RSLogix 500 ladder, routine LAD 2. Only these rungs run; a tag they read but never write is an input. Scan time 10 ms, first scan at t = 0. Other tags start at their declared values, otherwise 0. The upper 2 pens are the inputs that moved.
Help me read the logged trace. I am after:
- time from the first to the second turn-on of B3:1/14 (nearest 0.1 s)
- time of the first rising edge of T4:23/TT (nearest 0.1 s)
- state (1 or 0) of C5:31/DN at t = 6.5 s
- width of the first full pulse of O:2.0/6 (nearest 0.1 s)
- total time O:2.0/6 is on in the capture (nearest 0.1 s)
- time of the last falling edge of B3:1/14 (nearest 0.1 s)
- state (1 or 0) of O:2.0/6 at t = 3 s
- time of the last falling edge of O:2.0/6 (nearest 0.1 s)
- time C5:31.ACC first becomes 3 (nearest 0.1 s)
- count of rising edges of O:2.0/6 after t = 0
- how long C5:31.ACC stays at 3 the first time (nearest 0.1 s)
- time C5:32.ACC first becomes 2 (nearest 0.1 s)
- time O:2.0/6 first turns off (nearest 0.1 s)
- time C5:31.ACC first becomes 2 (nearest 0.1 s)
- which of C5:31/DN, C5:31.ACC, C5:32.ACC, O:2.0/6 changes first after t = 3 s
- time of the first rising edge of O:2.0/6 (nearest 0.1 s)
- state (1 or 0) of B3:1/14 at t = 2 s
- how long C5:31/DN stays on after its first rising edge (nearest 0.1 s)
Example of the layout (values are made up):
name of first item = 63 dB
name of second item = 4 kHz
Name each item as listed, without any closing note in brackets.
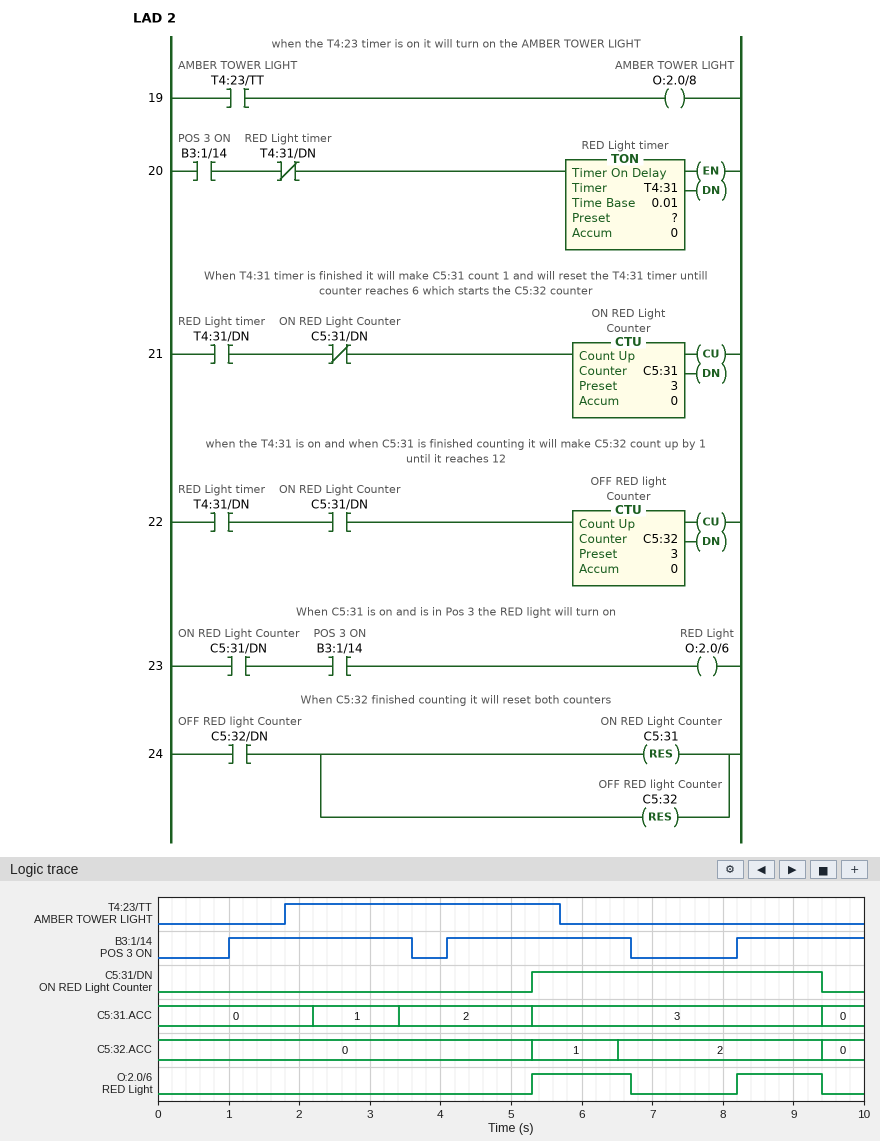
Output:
time from the first to the second turn-on of B3:1/14 = 3.1 s
time of the first rising edge of T4:23/TT = 1.8 s
state (1 or 0) of C5:31/DN at t = 6.5 s = 1
width of the first full pulse of O:2.0/6 = 1.4 s
total time O:2.0/6 is on in the capture = 2.6 s
time of the last falling edge of B3:1/14 = 6.7 s
state (1 or 0) of O:2.0/6 at t = 3 s = 0
time of the last falling edge of O:2.0/6 = 9.4 s
time C5:31.ACC first becomes 3 = 5.3 s
count of rising edges of O:2.0/6 after t = 0 = 2
how long C5:31.ACC stays at 3 the first time = 4.1 s
time C5:32.ACC first becomes 2 = 6.5 s
time O:2.0/6 first turns off = 6.7 s
time C5:31.ACC first becomes 2 = 3.4 s
which of C5:31/DN, C5:31.ACC, C5:32.ACC, O:2.0/6 changes first after t = 3 s = C5:31.ACC
time of the first rising edge of O:2.0/6 = 5.3 s
state (1 or 0) of B3:1/14 at t = 2 s = 1
how long C5:31/DN stays on after its first rising edge = 4.1 s
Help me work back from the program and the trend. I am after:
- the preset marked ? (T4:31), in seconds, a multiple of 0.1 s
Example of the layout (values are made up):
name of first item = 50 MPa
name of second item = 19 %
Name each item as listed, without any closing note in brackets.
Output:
the preset marked ? (T4:31), in seconds, a multiple of 0.1 s = 1.2 s
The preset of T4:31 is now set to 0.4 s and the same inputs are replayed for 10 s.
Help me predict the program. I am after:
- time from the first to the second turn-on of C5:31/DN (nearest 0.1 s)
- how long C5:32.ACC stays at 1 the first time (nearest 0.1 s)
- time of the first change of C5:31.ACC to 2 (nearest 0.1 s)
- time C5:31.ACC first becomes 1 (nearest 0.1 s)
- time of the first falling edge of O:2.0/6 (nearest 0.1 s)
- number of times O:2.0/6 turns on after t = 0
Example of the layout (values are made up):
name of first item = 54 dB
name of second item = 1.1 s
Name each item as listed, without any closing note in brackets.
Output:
time from the first to the second turn-on of C5:31/DN = 2.7 s
how long C5:32.ACC stays at 1 the first time = 0.4 s
time of the first change of C5:31.ACC to 2 = 1.8 s
time C5:31.ACC first becomes 1 = 1.4 s
time of the first falling edge of O:2.0/6 = 3.1 s
number of times O:2.0/6 turns on after t = 0 = 3
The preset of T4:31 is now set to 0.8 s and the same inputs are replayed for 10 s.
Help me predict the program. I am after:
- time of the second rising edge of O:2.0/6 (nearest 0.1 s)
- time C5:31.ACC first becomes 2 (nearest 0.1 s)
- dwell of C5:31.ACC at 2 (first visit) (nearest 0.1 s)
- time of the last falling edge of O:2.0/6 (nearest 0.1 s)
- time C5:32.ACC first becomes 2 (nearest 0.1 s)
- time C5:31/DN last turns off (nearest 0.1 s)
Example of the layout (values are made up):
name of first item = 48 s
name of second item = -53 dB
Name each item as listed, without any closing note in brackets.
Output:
time of the second rising edge of O:2.0/6 = 4.1 s
time C5:31.ACC first becomes 2 = 2.6 s
dwell of C5:31.ACC at 2 (first visit) = 0.8 s
time of the last falling edge of O:2.0/6 = 5.7 s
time C5:32.ACC first becomes 2 = 4.9 s
time C5:31/DN last turns off = 5.7 s
